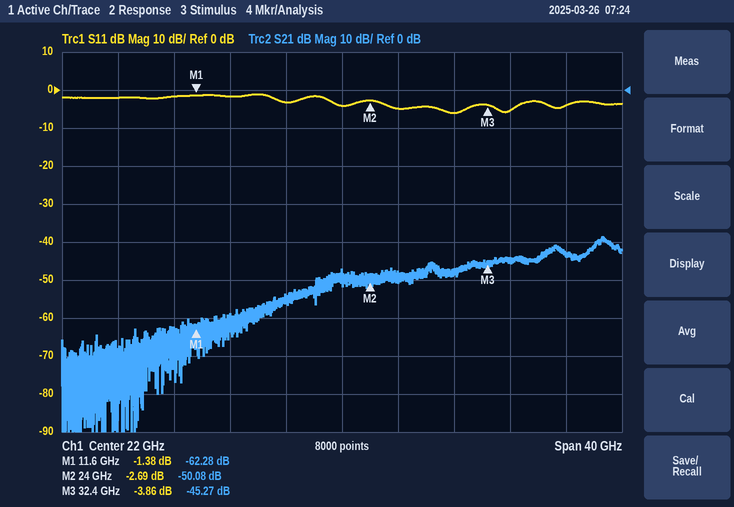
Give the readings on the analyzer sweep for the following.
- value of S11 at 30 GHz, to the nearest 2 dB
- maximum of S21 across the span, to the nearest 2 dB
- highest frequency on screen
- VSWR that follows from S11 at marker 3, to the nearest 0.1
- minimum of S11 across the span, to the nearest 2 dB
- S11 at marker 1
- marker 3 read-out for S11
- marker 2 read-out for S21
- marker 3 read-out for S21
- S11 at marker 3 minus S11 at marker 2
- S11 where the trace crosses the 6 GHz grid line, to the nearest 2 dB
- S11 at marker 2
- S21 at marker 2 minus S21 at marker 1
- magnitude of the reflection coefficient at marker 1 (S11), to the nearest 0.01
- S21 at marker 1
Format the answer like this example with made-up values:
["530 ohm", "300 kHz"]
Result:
["-6 dB", "-38 dB", "42 GHz", "4.6", "-6 dB", "-1.38 dB", "-3.86 dB", "-50.08 dB", "-45.27 dB", "-1.17 dB", "-2 dB", "-2.69 dB", "12.20 dB", "0.85", "-62.28 dB"]
